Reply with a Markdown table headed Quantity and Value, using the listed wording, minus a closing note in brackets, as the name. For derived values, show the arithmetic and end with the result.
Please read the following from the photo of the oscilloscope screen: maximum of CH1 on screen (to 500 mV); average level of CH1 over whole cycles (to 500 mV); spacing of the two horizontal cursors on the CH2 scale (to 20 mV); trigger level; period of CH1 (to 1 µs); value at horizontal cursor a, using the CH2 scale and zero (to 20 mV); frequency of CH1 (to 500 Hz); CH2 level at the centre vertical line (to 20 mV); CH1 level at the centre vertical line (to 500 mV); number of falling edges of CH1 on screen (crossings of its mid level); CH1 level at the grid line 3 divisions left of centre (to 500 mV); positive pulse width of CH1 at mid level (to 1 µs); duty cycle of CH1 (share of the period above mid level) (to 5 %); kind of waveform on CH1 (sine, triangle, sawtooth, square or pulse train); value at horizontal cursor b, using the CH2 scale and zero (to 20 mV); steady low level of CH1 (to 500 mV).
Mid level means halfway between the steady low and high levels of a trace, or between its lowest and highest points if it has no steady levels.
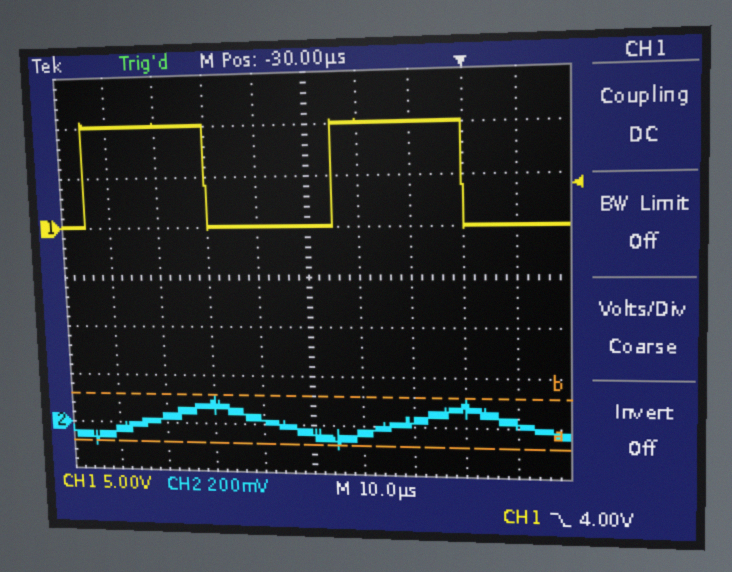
| Quantity | Value |
|---|---|
| maximum of CH1 on screen | 10.5 V |
| average level of CH1 over whole cycles | 0.0 V + 0.5 × (10.5 V − (0.0 V)) ≈ 5.25 V, so 5.0 V to the nearest 500 mV |
| spacing of the two horizontal cursors on the CH2 scale | 200 mV |
| trigger level | 4.00 V |
| period of CH1 | 50 µs |
| value at horizontal cursor a, using the CH2 scale and zero | -80 mV |
| frequency of CH1 | 1 / 50 µs ≈ 20.0 kHz |
| CH2 level at the centre vertical line | -40 mV |
| CH1 level at the centre vertical line | 0.0 V |
| number of falling edges of CH1 on screen | 2 |
| CH1 level at the grid line 3 divisions left of centre | 10.0 V |
| positive pulse width of CH1 at mid level | 25 µs |
| duty cycle of CH1 (share of the period above mid level) | 25 µs / 50 µs ≈ 50 % |
| kind of waveform on CH1 | square |
| value at horizontal cursor b, using the CH2 scale and zero | 120 mV |
| steady low level of CH1 | 0.0 V |
